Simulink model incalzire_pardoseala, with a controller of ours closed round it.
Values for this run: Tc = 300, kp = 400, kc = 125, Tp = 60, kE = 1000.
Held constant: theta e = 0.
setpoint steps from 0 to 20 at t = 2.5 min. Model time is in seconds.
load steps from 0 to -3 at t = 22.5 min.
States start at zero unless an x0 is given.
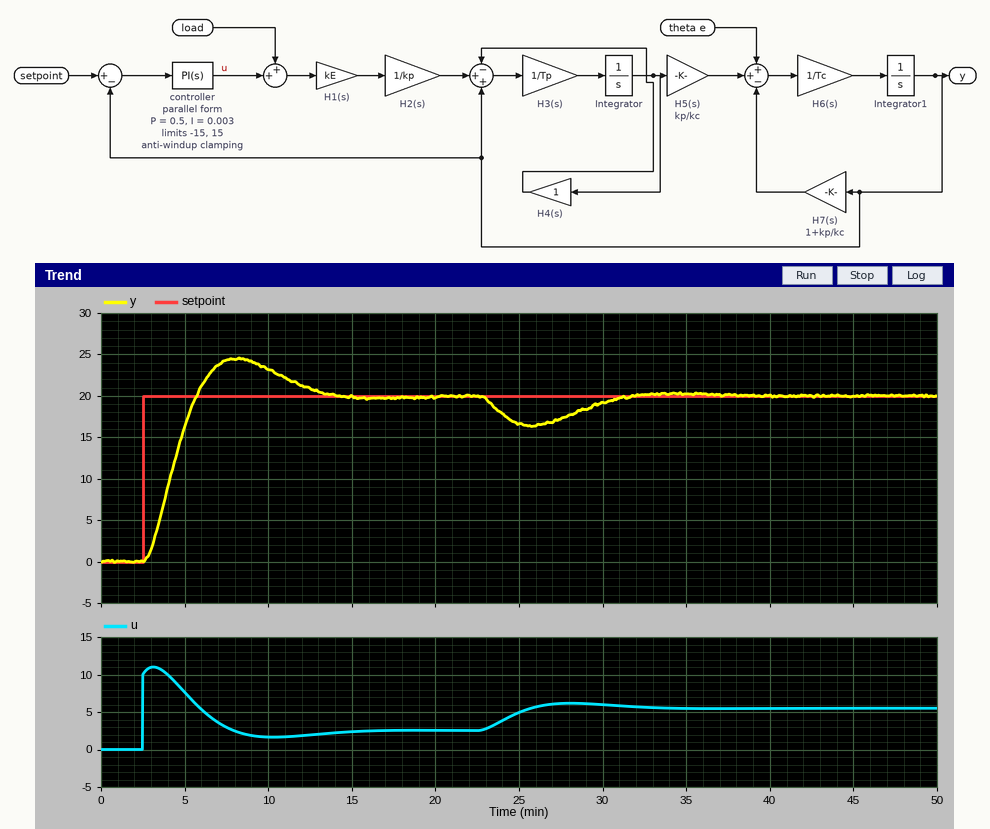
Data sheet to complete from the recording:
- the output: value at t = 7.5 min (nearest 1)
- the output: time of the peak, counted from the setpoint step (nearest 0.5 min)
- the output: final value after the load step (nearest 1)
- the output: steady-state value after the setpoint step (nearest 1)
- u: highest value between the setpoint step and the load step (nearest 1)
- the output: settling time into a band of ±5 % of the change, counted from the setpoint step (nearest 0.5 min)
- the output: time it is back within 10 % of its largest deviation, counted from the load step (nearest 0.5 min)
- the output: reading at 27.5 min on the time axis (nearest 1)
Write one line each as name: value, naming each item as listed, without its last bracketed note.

the output: value at t = 7.5 min: 24
the output: time of the peak, counted from the setpoint step: 5.5 min
the output: final value after the load step: 20
the output: steady-state value after the setpoint step: 20
u: highest value between the setpoint step and the load step: 11
the output: settling time into a band of ±5 % of the change, counted from the setpoint step: 10.0 min
the output: time it is back within 10 % of its largest deviation, counted from the load step: 8.5 min
the output: reading at 27.5 min on the time axis: 17
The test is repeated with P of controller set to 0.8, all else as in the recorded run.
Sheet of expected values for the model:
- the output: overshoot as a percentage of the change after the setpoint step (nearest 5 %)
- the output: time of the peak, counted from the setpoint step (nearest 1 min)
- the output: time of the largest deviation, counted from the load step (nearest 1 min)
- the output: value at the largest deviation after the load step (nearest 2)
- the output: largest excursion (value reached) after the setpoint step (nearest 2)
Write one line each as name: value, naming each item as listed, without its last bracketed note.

the output: overshoot as a percentage of the change after the setpoint step: 10 %
the output: time of the peak, counted from the setpoint step: 4 min
the output: time of the largest deviation, counted from the load step: 3 min
the output: value at the largest deviation after the load step: 18
the output: largest excursion (value reached) after the setpoint step: 22
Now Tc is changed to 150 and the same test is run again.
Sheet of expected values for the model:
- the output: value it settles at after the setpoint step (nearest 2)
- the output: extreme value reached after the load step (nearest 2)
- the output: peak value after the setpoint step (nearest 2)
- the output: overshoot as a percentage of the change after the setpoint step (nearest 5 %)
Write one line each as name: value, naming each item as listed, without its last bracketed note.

the output: value it settles at after the setpoint step: 20
the output: extreme value reached after the load step: 16
the output: peak value after the setpoint step: 22
the output: overshoot as a percentage of the change after the setpoint step: 15 %
